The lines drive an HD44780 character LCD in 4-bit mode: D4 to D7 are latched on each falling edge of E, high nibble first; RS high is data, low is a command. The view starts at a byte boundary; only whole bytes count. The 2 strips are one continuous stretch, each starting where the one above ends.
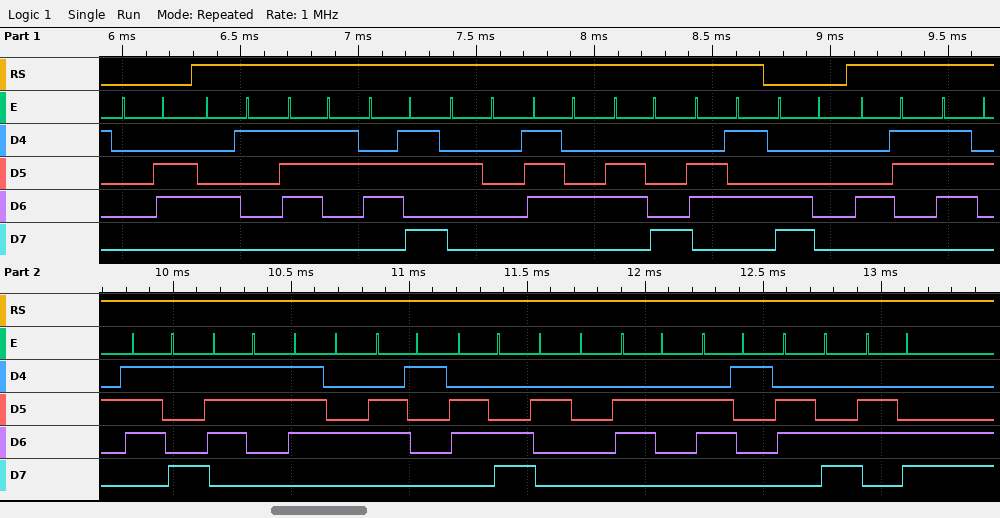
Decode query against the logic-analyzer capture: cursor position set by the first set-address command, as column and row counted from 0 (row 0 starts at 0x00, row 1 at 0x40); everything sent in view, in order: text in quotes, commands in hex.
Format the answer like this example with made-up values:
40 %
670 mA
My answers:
column 0, row 1
0x06 "Ask the" 0xC0 "Crystal ball"
